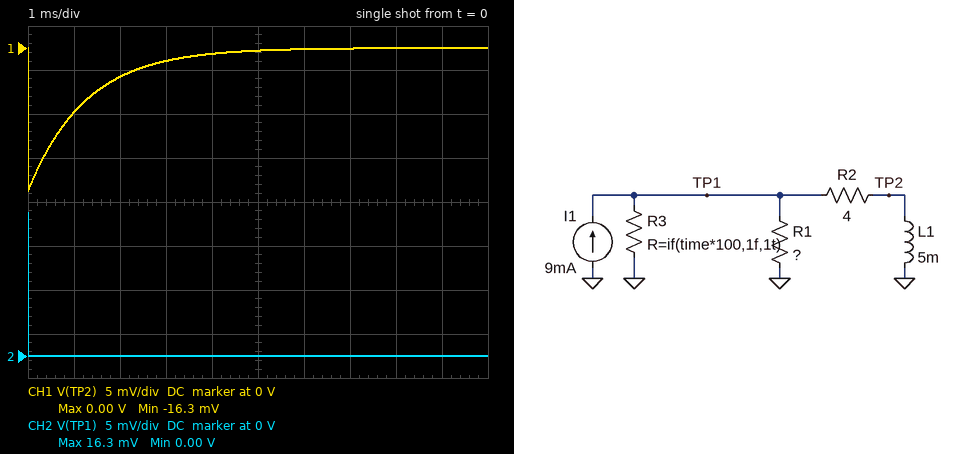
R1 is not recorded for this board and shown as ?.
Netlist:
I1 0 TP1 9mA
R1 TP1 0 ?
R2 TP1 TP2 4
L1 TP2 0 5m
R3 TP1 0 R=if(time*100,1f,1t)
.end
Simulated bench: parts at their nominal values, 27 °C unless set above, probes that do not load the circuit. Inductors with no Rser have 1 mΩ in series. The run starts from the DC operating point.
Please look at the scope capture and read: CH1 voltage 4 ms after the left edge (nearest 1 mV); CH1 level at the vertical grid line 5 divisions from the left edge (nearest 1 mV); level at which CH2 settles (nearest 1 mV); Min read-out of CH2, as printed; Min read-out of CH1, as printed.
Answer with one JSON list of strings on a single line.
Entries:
["-1 mV", "0 V", "0 V", "0.00 V", "-16.3 mV"]
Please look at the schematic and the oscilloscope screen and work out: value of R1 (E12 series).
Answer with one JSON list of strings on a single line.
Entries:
["3.3 Ω"]
